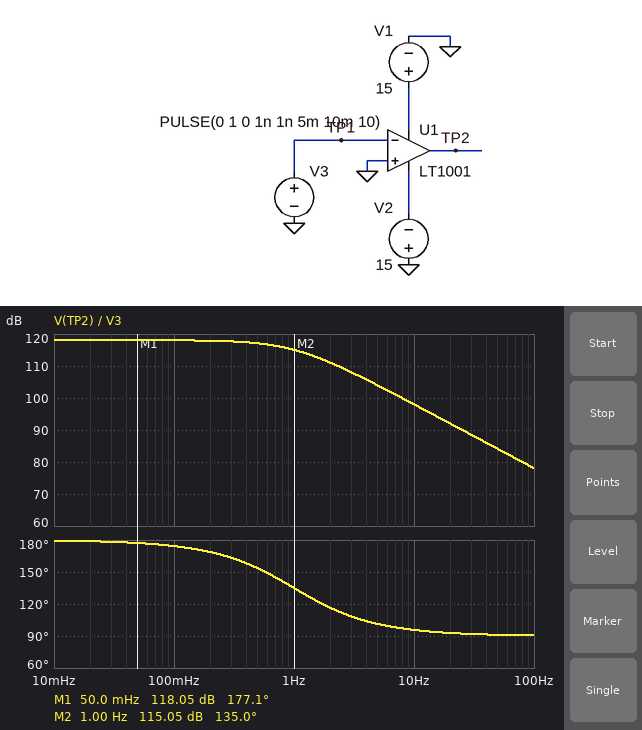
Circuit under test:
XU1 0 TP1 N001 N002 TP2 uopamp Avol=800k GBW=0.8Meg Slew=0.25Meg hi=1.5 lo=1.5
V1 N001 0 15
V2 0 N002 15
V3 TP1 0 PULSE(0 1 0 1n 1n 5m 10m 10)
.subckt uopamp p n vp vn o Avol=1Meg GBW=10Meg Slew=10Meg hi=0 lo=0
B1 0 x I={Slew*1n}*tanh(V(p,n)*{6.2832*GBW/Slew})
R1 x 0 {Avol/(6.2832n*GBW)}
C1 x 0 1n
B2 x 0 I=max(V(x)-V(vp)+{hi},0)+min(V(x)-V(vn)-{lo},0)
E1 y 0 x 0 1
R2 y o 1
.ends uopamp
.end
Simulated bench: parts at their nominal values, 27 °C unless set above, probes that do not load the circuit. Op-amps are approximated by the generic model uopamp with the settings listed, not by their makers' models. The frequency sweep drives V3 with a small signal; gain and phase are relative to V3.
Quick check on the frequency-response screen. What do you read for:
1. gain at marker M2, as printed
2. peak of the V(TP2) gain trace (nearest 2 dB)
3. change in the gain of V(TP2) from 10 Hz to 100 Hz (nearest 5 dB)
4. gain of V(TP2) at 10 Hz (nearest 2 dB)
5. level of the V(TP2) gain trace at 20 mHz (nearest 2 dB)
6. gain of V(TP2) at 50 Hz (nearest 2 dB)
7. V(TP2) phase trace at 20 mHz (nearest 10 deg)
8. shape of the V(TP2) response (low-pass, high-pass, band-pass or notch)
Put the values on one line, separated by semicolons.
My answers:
115.05 dB; 118 dB; -20 dB; 98 dB; 118 dB; 84 dB; 180 deg; low-pass
